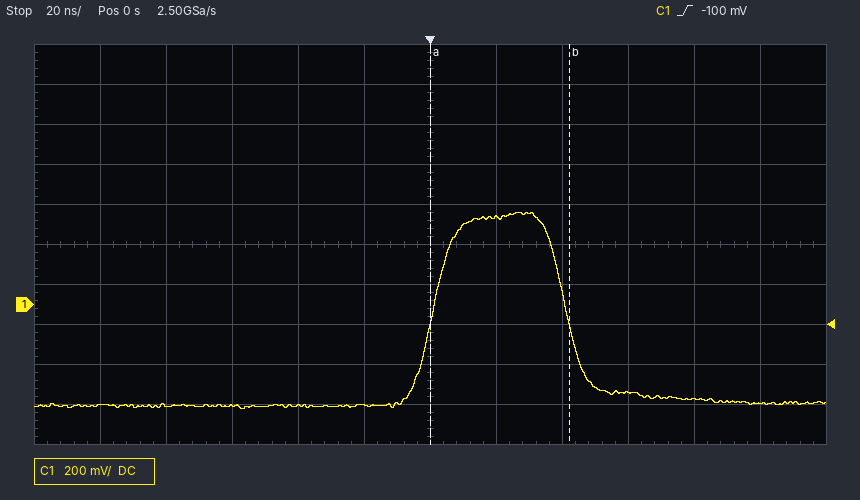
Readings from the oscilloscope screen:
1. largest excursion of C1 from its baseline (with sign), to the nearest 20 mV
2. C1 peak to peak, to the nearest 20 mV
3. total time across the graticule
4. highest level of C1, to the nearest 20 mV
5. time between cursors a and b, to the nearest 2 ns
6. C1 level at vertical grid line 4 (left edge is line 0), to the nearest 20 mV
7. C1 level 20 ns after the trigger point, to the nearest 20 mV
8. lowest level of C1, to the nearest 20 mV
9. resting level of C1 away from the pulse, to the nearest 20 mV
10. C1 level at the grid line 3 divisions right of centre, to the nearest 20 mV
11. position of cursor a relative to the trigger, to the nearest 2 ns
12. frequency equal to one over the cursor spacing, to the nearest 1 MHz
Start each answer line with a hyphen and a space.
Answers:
- +960 mV
- 980 mV
- 240 ns
- 460 mV
- 42 ns
- -500 mV
- 440 mV
- -520 mV
- -500 mV
- -440 mV
- 0 ns
- 24 MHz
